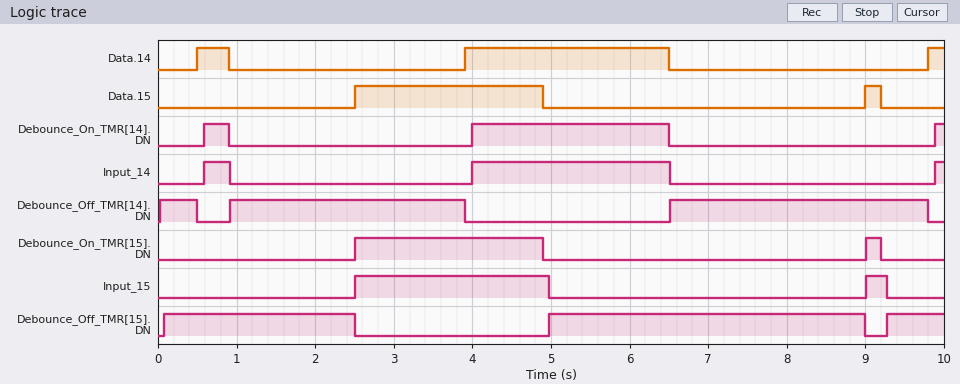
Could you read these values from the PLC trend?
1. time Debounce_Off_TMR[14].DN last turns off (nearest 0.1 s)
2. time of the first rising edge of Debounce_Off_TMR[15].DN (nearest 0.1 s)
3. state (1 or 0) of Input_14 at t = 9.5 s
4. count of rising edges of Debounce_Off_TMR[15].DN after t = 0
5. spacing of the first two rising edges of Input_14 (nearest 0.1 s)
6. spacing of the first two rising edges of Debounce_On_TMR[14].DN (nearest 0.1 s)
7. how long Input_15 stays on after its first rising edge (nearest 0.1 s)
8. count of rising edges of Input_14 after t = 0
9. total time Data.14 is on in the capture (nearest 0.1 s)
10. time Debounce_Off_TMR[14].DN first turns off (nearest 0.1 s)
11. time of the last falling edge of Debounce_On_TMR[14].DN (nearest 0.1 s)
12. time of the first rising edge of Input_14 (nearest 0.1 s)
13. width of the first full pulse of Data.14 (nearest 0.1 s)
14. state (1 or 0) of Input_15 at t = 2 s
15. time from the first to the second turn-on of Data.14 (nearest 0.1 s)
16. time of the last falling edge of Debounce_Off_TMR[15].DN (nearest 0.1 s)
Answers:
9.8 s
0.1 s
0
3
3.4 s
3.4 s
2.5 s
3
3.2 s
0.5 s
6.5 s
0.6 s
0.4 s
0
3.4 s
9.0 s
